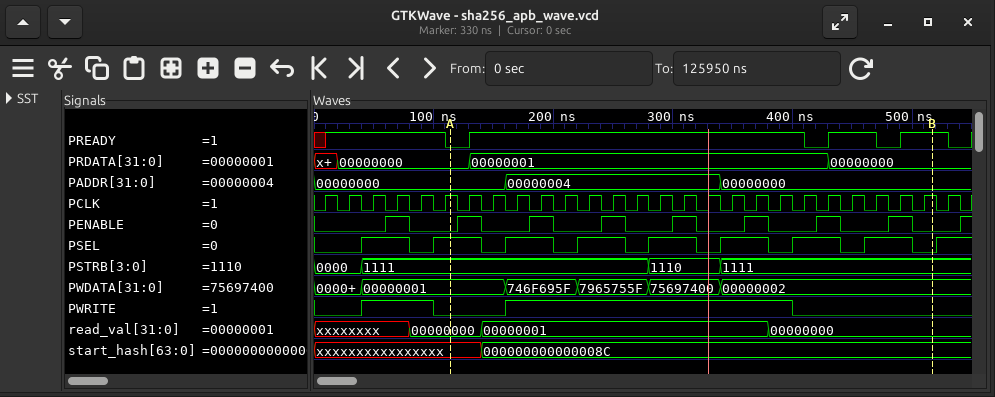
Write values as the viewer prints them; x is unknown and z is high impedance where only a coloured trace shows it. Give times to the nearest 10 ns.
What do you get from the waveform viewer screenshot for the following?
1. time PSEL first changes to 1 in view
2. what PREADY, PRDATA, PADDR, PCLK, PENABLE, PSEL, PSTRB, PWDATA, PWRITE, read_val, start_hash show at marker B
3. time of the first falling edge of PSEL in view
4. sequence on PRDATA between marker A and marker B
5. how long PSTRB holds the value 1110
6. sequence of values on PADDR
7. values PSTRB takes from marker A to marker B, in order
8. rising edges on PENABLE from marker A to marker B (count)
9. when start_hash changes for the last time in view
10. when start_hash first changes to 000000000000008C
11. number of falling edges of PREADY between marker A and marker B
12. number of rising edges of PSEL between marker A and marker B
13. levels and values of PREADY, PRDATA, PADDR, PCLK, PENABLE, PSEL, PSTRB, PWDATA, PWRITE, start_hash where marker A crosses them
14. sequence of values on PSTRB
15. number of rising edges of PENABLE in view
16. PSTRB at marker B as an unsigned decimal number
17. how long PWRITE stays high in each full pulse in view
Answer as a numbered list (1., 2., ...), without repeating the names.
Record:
1. 40 ns
2. PREADY=1, PRDATA=00000000, PADDR=00000000, PCLK=1, PENABLE=0, PSEL=0, PSTRB=1111, PWDATA=00000002, PWRITE=0, read_val=00000000, start_hash=000000000000008C
3. 80 ns
4. 00000000, 00000001, 00000000
5. 60 ns
6. 00000000, 00000004, 00000000
7. 1111, 1110, 1111
8. 7
9. 140 ns
10. 140 ns
11. 2
12. 6
13. PREADY=0, PRDATA=00000000, PADDR=00000000, PCLK=1, PENABLE=0, PSEL=1, PSTRB=1111, PWDATA=00000001, PWRITE=0, start_hash=xxxxxxxxxxxxxxxx
14. 0000, 1111, 1110, 1111
15. 9
16. 15
17. 60 ns, 240 ns
